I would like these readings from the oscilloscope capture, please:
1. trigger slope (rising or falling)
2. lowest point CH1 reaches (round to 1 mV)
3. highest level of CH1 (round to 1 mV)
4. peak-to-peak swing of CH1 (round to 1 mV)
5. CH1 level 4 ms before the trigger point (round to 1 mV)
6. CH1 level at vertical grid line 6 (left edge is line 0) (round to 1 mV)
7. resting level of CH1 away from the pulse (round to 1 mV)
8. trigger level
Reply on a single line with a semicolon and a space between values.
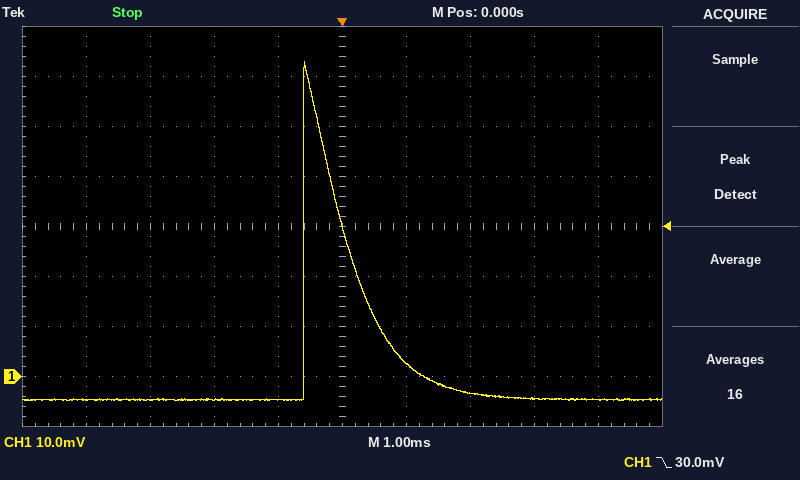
falling; -5 mV; 63 mV; 68 mV; -5 mV; 3 mV; -5 mV; 30.0 mV
